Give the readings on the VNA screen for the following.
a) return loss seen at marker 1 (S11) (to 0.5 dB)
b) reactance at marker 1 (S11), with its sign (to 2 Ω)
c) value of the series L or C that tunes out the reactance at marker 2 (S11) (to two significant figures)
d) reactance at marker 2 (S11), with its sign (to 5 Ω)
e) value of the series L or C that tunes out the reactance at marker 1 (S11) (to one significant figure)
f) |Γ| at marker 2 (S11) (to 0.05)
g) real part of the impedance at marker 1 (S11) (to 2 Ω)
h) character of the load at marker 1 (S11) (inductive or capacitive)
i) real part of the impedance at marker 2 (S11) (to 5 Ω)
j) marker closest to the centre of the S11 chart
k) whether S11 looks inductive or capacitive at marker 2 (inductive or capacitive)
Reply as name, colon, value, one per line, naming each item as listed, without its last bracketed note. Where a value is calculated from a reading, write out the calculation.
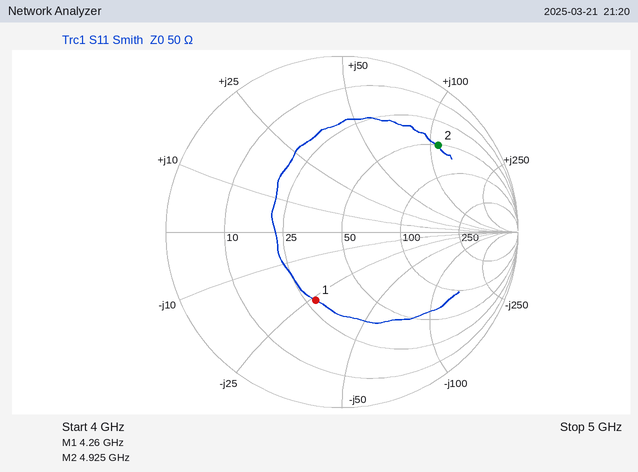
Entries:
return loss seen at marker 1 (S11): 7.5 dB
reactance at marker 1 (S11), with its sign: -26 Ω
value of the series L or C that tunes out the reactance at marker 2 (S11): C = 1/(2π × 4.925 GHz × 110 Ω) ≈ 294 fF, so 290 fF to two significant figures
reactance at marker 2 (S11), with its sign: +110 Ω
value of the series L or C that tunes out the reactance at marker 1 (S11): L = 26 Ω/(2π × 4.26 GHz) ≈ 1.0 nH
|Γ| at marker 2 (S11): 0.75
real part of the impedance at marker 1 (S11): 28 Ω
character of the load at marker 1 (S11): capacitive
real part of the impedance at marker 2 (S11): 50 Ω
marker closest to the centre of the S11 chart: marker 1
whether S11 looks inductive or capacitive at marker 2: inductive
